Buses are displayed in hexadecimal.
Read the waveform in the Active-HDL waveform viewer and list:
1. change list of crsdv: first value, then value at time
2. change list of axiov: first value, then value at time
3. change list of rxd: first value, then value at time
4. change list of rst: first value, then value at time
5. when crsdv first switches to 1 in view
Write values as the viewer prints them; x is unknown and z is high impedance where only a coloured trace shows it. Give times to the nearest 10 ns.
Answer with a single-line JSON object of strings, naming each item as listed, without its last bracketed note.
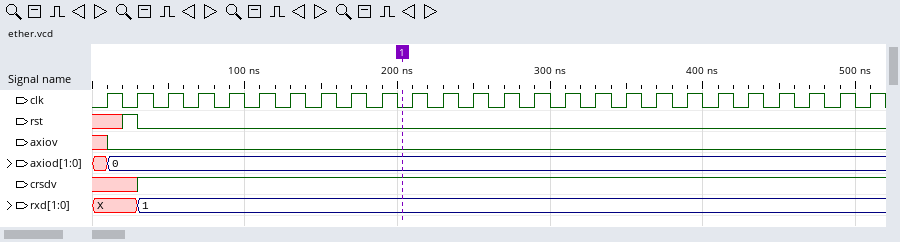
{"change list of crsdv: first value, then value at time": "x, 1 at 30 ns", "change list of axiov: first value, then value at time": "x, 0 at 10 ns", "change list of rxd: first value, then value at time": "X, 1 at 30 ns", "change list of rst: first value, then value at time": "x, 1 at 20 ns, 0 at 30 ns", "when crsdv first switches to 1 in view": "30 ns"}
